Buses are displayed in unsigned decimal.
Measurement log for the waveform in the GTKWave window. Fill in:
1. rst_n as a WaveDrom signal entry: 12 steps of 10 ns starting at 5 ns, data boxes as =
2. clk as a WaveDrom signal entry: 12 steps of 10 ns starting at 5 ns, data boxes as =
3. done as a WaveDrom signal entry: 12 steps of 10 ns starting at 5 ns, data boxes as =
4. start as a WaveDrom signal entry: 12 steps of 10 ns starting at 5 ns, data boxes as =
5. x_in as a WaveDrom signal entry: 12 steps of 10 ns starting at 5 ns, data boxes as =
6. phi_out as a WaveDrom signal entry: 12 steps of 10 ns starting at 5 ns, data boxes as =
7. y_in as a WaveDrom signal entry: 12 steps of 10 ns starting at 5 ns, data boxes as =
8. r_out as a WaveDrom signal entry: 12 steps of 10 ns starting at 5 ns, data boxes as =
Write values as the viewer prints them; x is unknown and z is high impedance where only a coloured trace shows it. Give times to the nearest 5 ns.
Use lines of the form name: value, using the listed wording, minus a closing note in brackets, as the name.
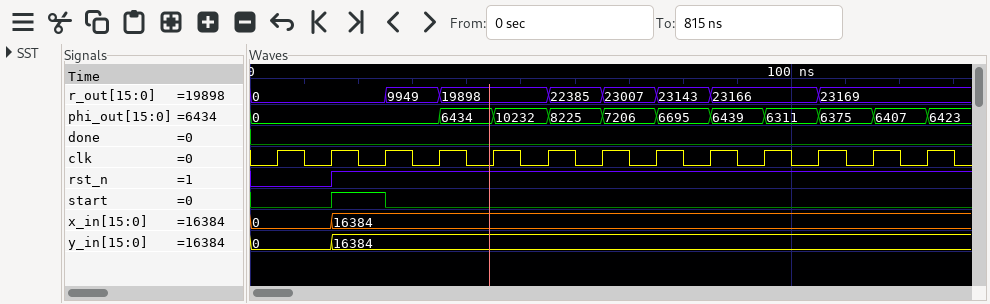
rst_n as a WaveDrom signal entry: 12 steps of 10 ns starting at 5 ns, data boxes as =: {name: 'rst_n', wave: '01..........'}
clk as a WaveDrom signal entry: 12 steps of 10 ns starting at 5 ns, data boxes as =: {name: 'clk', wave: 'p...........'}
done as a WaveDrom signal entry: 12 steps of 10 ns starting at 5 ns, data boxes as =: {name: 'done', wave: '0...........'}
start as a WaveDrom signal entry: 12 steps of 10 ns starting at 5 ns, data boxes as =: {name: 'start', wave: '010.........'}
x_in as a WaveDrom signal entry: 12 steps of 10 ns starting at 5 ns, data boxes as =: {name: 'x_in', wave: '==..........', data: '0 16384'}
phi_out as a WaveDrom signal entry: 12 steps of 10 ns starting at 5 ns, data boxes as =: {name: 'phi_out', wave: '=..=========', data: '0 6434 10232 8225 7206 6695 6439 6311 6375 6407'}
y_in as a WaveDrom signal entry: 12 steps of 10 ns starting at 5 ns, data boxes as =: {name: 'y_in', wave: '==..........', data: '0 16384'}
r_out as a WaveDrom signal entry: 12 steps of 10 ns starting at 5 ns, data boxes as =: {name: 'r_out', wave: '=.==.====.=.', data: '0 9949 19898 22385 23007 23143 23166 23169'}
